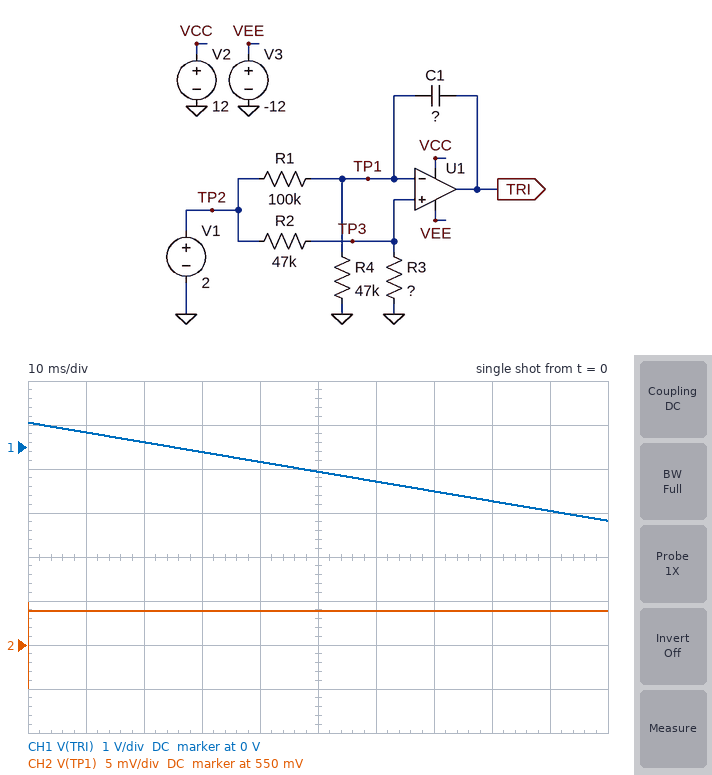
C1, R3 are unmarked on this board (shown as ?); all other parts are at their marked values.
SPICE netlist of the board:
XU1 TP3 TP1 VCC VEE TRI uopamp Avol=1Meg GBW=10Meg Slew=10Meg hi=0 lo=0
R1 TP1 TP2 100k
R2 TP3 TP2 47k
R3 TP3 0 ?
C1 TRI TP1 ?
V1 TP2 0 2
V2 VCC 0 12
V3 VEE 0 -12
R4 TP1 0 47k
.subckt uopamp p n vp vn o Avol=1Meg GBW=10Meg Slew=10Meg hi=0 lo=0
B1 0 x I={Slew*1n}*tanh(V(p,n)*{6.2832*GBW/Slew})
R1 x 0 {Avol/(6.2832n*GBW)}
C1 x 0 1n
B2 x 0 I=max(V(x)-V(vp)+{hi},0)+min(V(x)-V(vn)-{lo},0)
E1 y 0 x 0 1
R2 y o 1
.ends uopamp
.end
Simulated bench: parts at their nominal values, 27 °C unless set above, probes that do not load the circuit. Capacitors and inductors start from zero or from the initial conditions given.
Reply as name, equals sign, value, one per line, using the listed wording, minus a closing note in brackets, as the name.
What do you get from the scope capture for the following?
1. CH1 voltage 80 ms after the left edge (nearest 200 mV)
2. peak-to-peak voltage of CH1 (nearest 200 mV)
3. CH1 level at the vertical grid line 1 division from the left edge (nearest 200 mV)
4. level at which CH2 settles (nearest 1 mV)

CH1 voltage 80 ms after the left edge = -1.2 V
peak-to-peak voltage of CH1 = 2.2 V
CH1 level at the vertical grid line 1 division from the left edge = 400 mV
level at which CH2 settles = 554 mV
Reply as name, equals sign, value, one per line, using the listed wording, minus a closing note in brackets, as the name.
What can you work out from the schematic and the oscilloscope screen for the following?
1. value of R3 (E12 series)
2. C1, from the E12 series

value of R3 = 18 kΩ
C1, from the E12 series = 120 nF
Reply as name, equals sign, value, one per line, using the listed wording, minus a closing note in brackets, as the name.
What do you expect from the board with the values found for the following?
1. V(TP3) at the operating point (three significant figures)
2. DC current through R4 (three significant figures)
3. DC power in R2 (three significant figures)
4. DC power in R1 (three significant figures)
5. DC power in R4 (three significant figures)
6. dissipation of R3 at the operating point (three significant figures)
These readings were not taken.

V(TP3) at the operating point = 554 mV
DC current through R4 = 13.6 µA
DC power in R2 = 44.5 µW
DC power in R1 = 18.5 µW
DC power in R4 = 8.70 µW
dissipation of R3 at the operating point = 17.0 µW
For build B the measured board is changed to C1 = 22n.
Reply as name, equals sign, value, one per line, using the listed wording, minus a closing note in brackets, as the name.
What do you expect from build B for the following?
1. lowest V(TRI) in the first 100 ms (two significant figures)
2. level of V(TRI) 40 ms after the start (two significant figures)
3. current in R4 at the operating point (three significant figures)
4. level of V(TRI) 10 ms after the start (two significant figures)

lowest V(TRI) in the first 100 ms = -12 V
level of V(TRI) 40 ms after the start = -4.3 V
current in R4 at the operating point = 13.6 µA
level of V(TRI) 10 ms after the start = -660 mV
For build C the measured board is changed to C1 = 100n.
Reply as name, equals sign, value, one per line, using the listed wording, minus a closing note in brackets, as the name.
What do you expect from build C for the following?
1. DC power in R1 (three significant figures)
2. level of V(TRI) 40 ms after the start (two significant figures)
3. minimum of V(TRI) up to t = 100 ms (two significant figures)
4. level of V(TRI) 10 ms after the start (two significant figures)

DC power in R1 = 18.5 µW
level of V(TRI) 40 ms after the start = -520 mV
minimum of V(TRI) up to t = 100 ms = -2.1 V
level of V(TRI) 10 ms after the start = 290 mV
